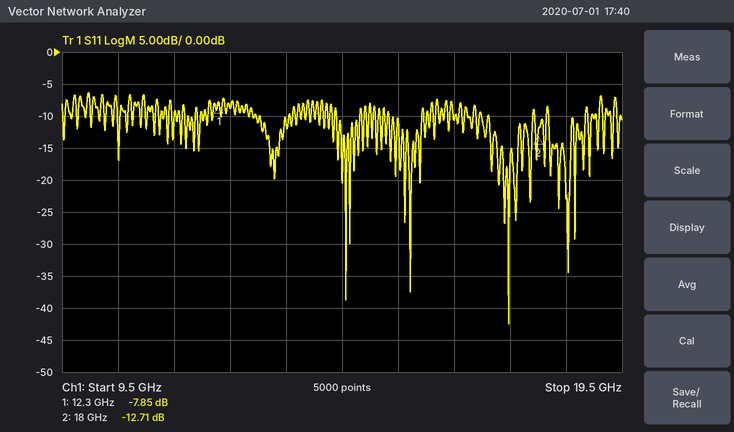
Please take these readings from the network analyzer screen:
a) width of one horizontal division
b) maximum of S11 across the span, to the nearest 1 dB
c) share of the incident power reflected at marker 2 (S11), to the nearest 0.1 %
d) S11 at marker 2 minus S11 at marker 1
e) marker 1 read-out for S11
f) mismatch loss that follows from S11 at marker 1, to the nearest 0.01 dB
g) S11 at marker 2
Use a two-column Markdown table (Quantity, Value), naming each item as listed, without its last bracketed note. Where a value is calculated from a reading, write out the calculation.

| Quantity | Value |
|---|---|
| width of one horizontal division | 1 GHz |
| maximum of S11 across the span, to the nearest 1 dB | -6 dB |
| share of the incident power reflected at marker 2 (S11), to the nearest 0.1 % | 10^(-12.71/10) ≈ 5.4 % |
| S11 at marker 2 minus S11 at marker 1 | -12.71 − (-7.85) = -4.86 dB |
| marker 1 read-out for S11 | -7.85 dB |
| mismatch loss that follows from S11 at marker 1, to the nearest 0.01 dB | −10 log10(1 − 10^(-7.85/10)) ≈ 0.78 dB |
| S11 at marker 2 | -12.71 dB |
